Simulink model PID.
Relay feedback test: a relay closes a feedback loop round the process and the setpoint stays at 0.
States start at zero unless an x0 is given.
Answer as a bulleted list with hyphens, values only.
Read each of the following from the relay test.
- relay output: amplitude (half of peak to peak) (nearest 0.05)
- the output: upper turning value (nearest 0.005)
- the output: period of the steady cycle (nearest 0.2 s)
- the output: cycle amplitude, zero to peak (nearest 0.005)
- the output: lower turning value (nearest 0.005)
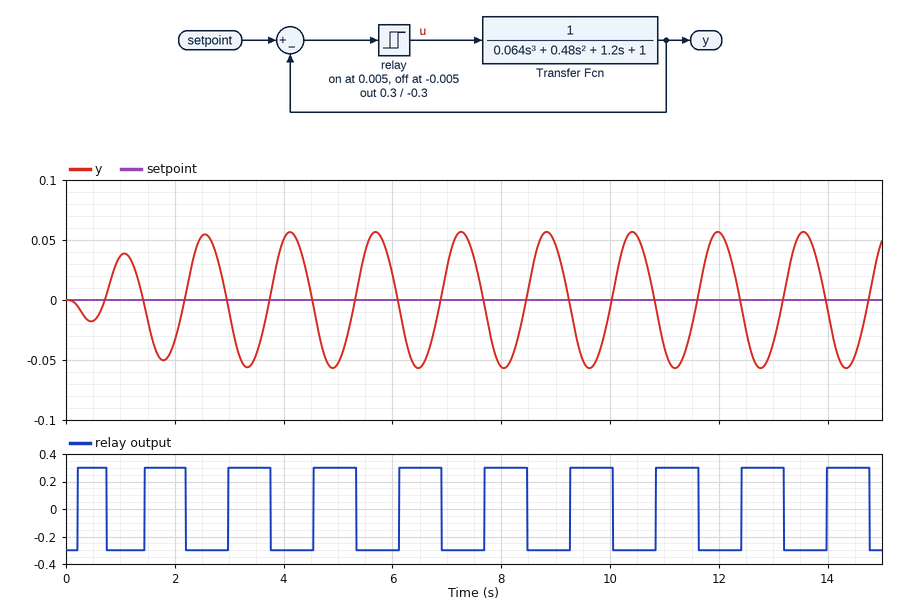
- 0.30
- 0.055
- 1.6 s
- 0.055
- -0.055
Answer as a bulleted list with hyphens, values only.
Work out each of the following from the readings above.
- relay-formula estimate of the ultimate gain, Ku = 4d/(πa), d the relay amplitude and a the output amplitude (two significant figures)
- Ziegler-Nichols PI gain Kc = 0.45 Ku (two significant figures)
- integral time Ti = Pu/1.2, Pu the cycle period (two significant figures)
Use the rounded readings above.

- 6.9
- 3.1
- 1.3 s
